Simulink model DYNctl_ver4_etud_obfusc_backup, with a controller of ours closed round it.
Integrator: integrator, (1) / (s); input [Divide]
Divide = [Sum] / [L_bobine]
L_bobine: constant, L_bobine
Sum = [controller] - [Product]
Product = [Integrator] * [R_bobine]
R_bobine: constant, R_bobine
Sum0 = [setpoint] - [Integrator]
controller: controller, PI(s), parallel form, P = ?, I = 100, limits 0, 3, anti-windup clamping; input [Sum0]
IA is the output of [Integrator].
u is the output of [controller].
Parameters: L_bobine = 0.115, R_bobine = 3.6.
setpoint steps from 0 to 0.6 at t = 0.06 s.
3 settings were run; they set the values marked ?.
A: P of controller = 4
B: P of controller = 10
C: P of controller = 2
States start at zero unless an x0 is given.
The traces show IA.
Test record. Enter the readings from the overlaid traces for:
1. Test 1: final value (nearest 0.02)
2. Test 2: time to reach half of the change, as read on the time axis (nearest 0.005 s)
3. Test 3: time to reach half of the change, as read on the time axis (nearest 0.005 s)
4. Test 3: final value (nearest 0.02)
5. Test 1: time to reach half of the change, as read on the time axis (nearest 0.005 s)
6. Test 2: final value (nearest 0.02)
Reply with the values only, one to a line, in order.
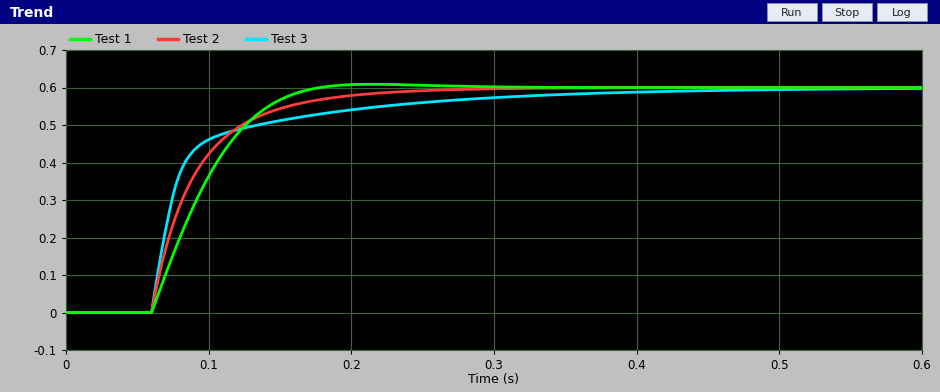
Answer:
0.60
0.080 s
0.075 s
0.60
0.090 s
0.60
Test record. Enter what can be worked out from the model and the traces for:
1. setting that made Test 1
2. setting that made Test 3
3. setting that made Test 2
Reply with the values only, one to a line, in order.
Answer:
C
B
A
